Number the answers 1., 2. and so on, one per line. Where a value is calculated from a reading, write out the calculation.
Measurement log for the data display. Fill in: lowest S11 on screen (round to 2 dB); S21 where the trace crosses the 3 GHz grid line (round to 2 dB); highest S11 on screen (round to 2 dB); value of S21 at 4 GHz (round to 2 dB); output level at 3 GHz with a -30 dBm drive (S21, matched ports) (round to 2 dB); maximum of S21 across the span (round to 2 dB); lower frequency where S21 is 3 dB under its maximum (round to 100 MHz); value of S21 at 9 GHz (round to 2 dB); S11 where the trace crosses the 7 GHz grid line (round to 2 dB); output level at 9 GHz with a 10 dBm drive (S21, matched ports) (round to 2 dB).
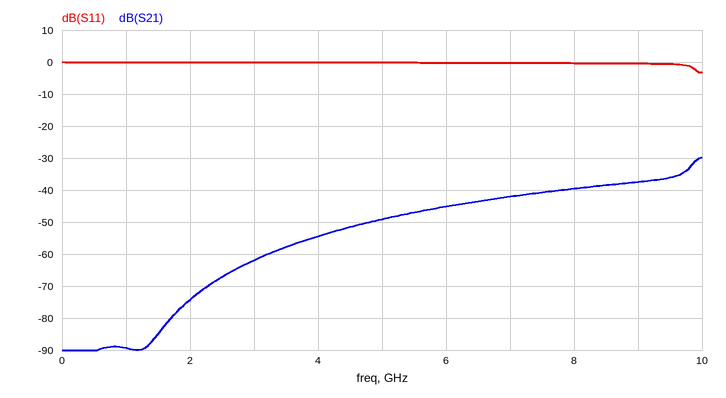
1. -4 dB
2. -62 dB
3. 0 dB
4. -54 dB
5. -30 dBm + (-62 dB) = -92 dBm
6. -30 dB
7. 9.8 GHz
8. -38 dB
9. 0 dB
10. 10 dBm + (-38 dB) = -28 dBm
